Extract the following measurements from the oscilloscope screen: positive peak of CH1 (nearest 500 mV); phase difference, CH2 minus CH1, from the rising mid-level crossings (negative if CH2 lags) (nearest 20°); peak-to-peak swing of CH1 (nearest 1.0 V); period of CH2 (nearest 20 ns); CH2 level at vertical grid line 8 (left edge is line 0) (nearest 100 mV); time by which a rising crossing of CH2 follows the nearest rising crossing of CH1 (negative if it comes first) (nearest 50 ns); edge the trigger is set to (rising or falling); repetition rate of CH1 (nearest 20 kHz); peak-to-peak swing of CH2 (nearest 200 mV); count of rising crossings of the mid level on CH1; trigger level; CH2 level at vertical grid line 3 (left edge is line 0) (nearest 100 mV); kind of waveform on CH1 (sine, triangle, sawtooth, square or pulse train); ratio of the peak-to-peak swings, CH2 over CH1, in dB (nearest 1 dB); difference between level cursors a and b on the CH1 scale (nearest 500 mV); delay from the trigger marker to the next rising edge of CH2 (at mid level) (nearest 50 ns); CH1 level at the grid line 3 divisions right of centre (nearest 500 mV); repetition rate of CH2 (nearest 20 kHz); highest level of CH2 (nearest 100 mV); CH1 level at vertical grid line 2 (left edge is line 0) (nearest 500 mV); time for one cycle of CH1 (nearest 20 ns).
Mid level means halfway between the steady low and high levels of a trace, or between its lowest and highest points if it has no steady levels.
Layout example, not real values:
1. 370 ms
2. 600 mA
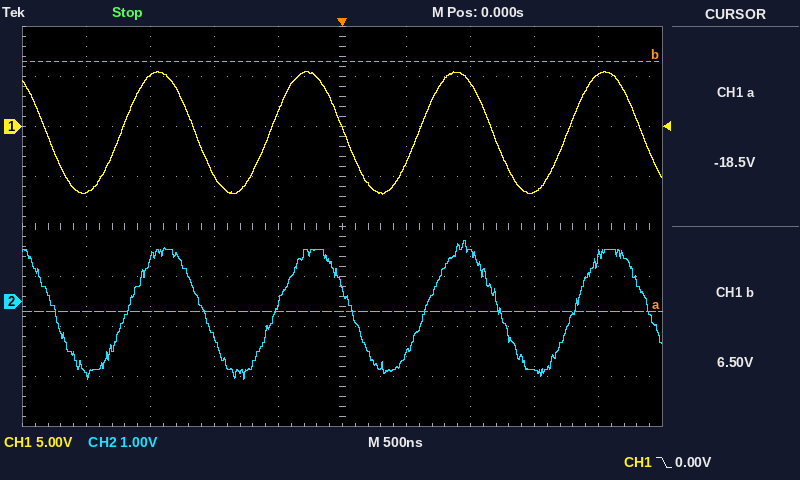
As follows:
1. 5.5 V
2. -20°
3. 12.0 V
4. 1.16 µs
5. -1.4 V
6. +50 ns
7. falling
8. 860 kHz
9. 2.8 V
10. 4
11. 0.00 V
12. -700 mV
13. sine
14. -13 dB
15. 25.0 V
16. 650 ns
17. -6.5 V
18. 860 kHz
19. 1.2 V
20. 5.0 V
21. 1.16 µs
